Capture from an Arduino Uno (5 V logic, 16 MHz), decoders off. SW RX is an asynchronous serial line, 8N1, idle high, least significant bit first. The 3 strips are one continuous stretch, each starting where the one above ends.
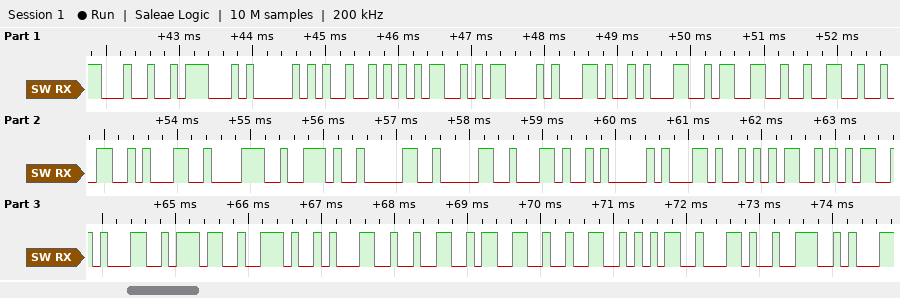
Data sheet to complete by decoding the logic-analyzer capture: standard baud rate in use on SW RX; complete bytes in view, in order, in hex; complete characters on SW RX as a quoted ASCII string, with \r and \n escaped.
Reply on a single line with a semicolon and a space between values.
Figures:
9600 baud; 0x24 0x47 0x50 0x52 0x4D 0x43 0x2C 0x31 0x33 0x32 0x32 0x31 0x38 0x2E 0x30 0x30 0x2C 0x41 0x2C 0x35 0x35 0x31 0x37 0x2E 0x31 0x32 0x33 0x32 0x35 0x2C 0x4E; "$GPRMC,132218.00,A,5517.12325,N"
